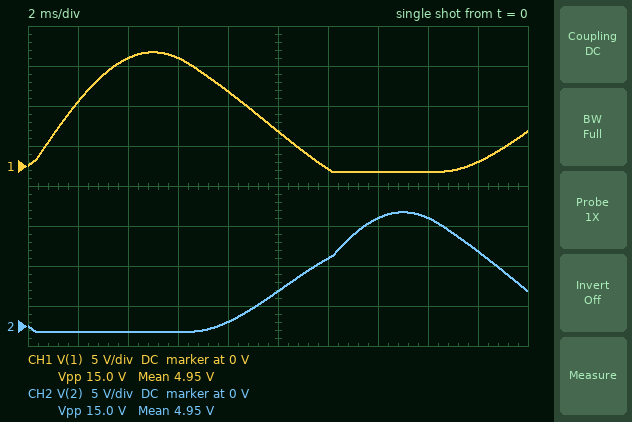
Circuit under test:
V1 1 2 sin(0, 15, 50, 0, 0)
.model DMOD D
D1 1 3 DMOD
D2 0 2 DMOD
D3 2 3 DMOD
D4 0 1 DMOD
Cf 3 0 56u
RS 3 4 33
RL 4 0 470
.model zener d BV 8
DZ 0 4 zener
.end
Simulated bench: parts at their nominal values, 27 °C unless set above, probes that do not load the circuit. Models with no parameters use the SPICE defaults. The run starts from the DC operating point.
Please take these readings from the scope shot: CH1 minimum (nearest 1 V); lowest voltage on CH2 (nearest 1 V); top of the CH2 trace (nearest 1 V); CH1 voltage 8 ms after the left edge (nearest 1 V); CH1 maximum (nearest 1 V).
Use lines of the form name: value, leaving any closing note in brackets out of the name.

CH1 minimum: -1 V
lowest voltage on CH2: -1 V
top of the CH2 trace: 14 V
CH1 voltage 8 ms after the left edge: 9 V
CH1 maximum: 14 V
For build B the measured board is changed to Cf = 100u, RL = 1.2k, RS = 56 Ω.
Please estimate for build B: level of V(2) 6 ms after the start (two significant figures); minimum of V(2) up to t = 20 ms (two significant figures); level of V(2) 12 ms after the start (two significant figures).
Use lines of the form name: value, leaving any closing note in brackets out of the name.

level of V(2) 6 ms after the start: -660 mV
minimum of V(2) up to t = 20 ms: -810 mV
level of V(2) 12 ms after the start: 9.3 V
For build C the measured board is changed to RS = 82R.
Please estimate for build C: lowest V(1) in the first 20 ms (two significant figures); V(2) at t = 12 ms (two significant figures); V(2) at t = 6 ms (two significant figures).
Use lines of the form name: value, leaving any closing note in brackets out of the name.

lowest V(1) in the first 20 ms: -790 mV
V(2) at t = 12 ms: 9.1 V
V(2) at t = 6 ms: -680 mV
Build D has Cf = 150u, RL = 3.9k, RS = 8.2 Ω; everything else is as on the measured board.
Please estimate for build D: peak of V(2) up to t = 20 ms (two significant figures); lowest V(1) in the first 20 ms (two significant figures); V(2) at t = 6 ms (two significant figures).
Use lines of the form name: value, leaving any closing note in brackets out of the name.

peak of V(2) up to t = 20 ms: 14 V
lowest V(1) in the first 20 ms: -830 mV
V(2) at t = 6 ms: -810 mV
